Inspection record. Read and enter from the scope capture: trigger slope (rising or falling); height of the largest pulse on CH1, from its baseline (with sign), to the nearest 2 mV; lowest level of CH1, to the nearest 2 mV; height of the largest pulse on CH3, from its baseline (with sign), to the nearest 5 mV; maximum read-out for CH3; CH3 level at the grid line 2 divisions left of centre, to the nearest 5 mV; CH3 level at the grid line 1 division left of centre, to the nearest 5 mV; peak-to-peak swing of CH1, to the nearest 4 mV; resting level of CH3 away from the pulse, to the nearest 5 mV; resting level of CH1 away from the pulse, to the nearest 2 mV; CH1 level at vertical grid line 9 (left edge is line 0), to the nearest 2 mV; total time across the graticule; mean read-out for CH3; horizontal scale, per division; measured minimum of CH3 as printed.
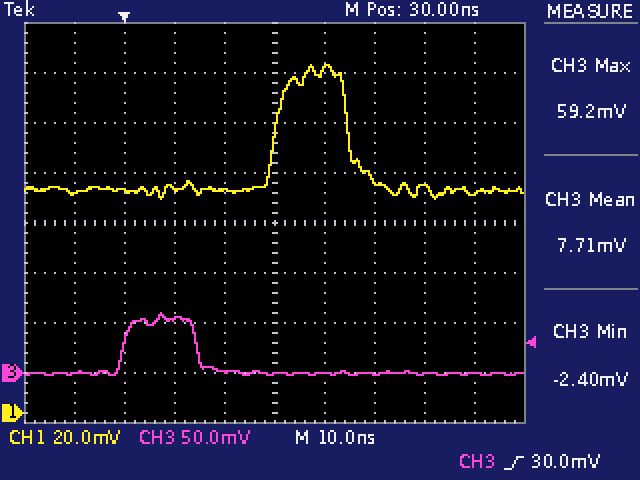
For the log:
rising
+50 mV
86 mV
+60 mV
59.2 mV
55 mV
0 mV
52 mV
0 mV
90 mV
88 mV
100 ns
7.71 mV
10 ns
-2.40 mV
